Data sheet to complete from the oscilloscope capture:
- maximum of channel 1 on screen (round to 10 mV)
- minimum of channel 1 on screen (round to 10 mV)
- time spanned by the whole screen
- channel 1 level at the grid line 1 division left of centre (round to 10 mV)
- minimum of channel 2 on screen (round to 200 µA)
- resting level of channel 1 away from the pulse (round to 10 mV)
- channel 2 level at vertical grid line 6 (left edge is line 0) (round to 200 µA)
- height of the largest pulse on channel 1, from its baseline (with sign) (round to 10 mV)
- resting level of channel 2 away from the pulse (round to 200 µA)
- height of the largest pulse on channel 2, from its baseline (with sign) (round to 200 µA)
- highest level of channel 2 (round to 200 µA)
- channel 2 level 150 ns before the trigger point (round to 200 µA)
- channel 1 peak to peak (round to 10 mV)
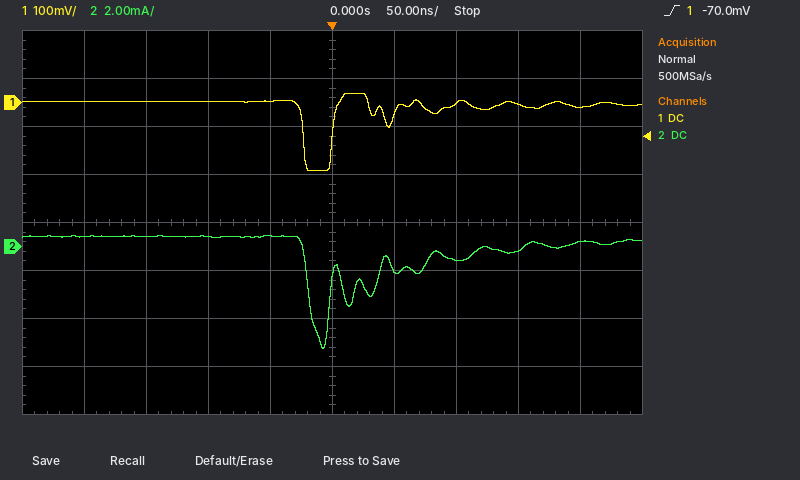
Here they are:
20 mV
-140 mV
500 ns
0 mV
-4.2 mA
0 mV
-1.0 mA
-140 mV
400 µA
-4.6 mA
400 µA
400 µA
160 mV
